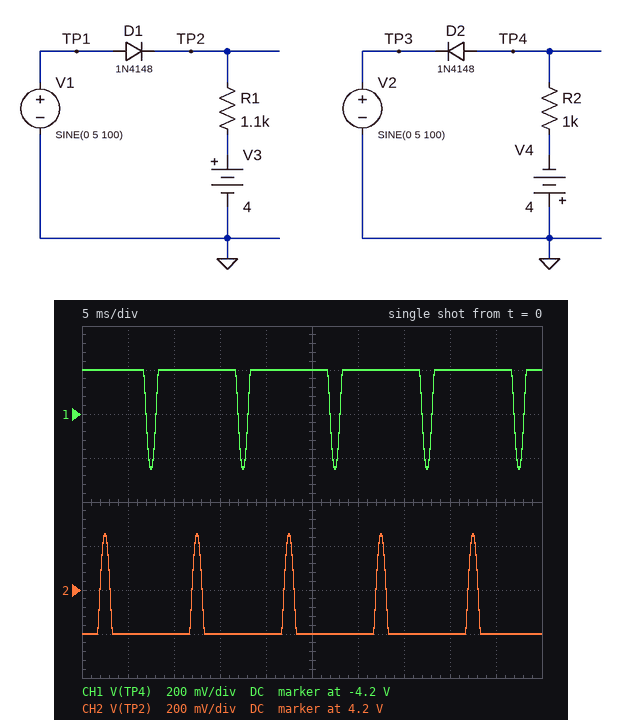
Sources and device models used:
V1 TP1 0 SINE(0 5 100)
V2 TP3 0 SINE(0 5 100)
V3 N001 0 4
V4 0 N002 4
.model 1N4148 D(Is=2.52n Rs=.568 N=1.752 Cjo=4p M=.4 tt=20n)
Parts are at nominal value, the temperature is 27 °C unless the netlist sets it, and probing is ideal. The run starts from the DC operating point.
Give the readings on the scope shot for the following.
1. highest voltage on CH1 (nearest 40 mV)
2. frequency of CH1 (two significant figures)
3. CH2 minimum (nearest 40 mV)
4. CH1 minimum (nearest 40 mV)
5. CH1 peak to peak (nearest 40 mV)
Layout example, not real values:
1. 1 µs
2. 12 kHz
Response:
1. -4.00 V
2. 100 Hz
3. 4.00 V
4. -4.44 V
5. 440 mV
